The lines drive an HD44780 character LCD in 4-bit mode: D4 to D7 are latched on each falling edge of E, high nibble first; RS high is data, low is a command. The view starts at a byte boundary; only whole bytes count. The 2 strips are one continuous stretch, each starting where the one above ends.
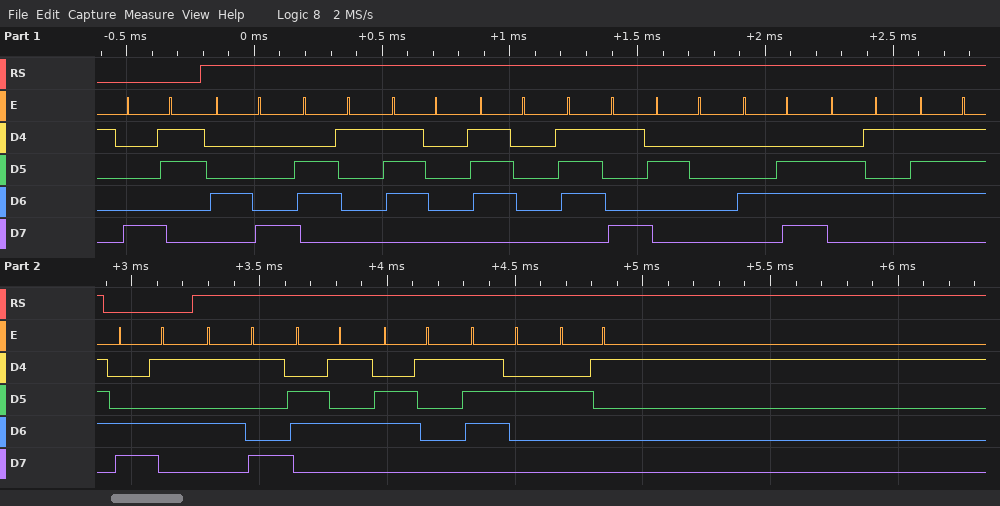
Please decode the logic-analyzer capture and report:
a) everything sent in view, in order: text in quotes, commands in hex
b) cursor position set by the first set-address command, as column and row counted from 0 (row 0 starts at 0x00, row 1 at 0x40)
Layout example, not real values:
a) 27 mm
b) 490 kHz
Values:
a) 0x83 "Happy New" 0xC5 "Year!"
b) column 3, row 0
